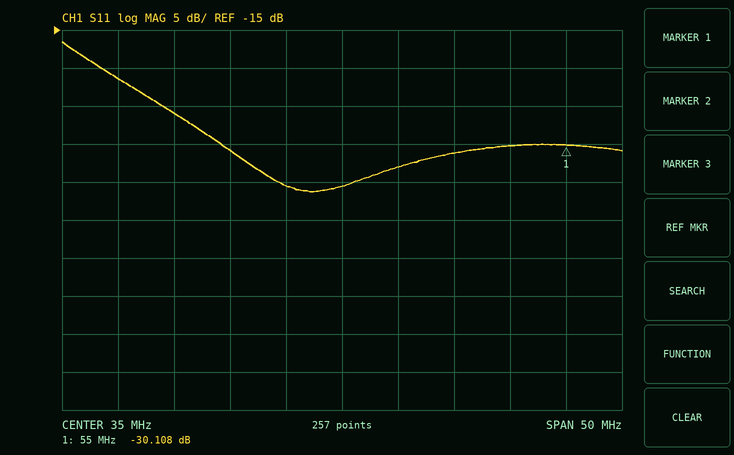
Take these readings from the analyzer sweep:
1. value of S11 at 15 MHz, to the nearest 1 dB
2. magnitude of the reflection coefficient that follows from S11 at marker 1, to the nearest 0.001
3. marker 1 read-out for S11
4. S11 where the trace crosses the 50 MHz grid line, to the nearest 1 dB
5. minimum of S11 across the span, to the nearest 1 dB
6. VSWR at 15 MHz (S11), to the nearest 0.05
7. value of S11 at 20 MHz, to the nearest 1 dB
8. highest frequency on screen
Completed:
-21 dB
0.031
-30.108 dB
-30 dB
-36 dB
1.20
-26 dB
60 MHz
